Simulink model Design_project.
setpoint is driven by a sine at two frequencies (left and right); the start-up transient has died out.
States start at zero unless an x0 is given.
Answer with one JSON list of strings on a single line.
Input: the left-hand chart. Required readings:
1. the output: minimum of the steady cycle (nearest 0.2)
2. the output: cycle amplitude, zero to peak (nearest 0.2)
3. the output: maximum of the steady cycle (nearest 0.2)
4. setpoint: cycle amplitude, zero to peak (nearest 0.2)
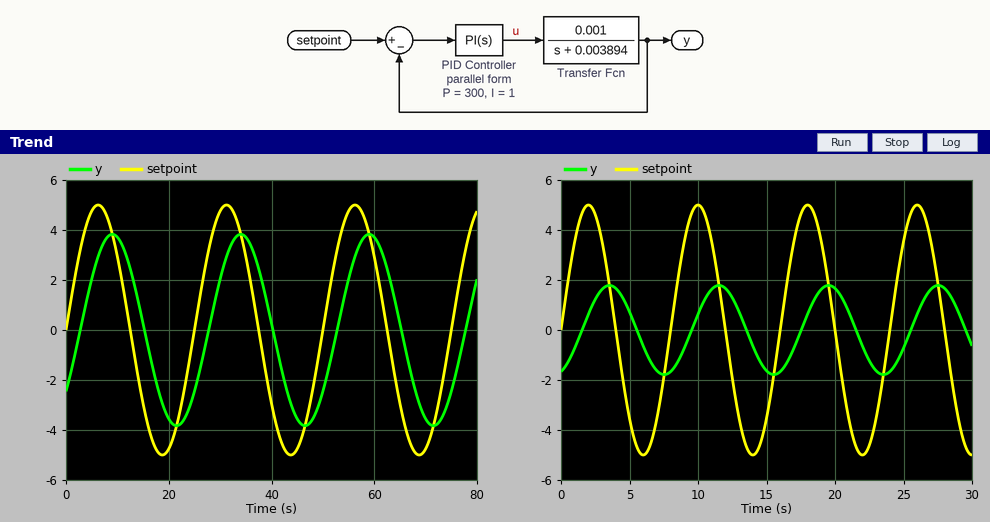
["-3.8", "3.8", "3.8", "5.0"]
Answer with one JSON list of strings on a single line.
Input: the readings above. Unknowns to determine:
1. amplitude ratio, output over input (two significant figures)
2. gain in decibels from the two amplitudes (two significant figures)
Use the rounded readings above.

["0.76", "-2.4 dB"]
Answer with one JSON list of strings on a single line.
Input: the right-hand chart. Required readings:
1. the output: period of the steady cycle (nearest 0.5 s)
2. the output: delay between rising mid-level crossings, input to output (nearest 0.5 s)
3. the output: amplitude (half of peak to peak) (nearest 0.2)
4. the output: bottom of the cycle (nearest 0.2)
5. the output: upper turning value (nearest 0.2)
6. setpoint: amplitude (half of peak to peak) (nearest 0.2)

["8.0 s", "1.5 s", "1.8", "-1.8", "1.8", "5.0"]
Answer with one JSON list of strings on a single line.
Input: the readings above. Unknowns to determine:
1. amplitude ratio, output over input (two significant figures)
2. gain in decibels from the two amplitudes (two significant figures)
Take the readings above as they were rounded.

["0.36", "-8.9 dB"]
